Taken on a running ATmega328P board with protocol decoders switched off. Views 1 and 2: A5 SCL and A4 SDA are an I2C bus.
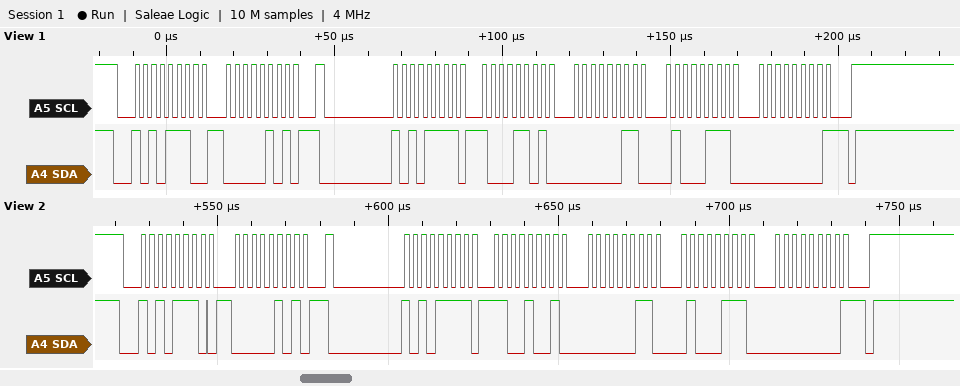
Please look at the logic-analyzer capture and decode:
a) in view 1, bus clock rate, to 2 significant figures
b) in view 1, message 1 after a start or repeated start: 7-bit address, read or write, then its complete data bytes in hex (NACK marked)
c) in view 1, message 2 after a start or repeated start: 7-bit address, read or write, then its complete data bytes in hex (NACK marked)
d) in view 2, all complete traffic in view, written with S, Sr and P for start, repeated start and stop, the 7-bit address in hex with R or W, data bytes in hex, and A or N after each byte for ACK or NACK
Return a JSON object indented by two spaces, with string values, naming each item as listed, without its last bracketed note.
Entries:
{
  "in view 1, bus clock rate, to 2 significant figures": "400 kHz",
  "in view 1, message 1 after a start or repeated start: 7-bit address, read or write, then its complete data bytes in hex": "0x57 write: 05",
  "in view 1, message 2 after a start or repeated start: 7-bit address, read or write, then its complete data bytes in hex": "0x57 read: 8D 03 47 00 NACK",
  "in view 2, all complete traffic in view, written with S, Sr and P for start, repeated start and stop, the 7-bit address in hex with R or W, data bytes in hex, and A or N after each byte for ACK or NACK": "S 57W A 05 A Sr 57R A C9 A 03 A 47 A 00 N P"
}
